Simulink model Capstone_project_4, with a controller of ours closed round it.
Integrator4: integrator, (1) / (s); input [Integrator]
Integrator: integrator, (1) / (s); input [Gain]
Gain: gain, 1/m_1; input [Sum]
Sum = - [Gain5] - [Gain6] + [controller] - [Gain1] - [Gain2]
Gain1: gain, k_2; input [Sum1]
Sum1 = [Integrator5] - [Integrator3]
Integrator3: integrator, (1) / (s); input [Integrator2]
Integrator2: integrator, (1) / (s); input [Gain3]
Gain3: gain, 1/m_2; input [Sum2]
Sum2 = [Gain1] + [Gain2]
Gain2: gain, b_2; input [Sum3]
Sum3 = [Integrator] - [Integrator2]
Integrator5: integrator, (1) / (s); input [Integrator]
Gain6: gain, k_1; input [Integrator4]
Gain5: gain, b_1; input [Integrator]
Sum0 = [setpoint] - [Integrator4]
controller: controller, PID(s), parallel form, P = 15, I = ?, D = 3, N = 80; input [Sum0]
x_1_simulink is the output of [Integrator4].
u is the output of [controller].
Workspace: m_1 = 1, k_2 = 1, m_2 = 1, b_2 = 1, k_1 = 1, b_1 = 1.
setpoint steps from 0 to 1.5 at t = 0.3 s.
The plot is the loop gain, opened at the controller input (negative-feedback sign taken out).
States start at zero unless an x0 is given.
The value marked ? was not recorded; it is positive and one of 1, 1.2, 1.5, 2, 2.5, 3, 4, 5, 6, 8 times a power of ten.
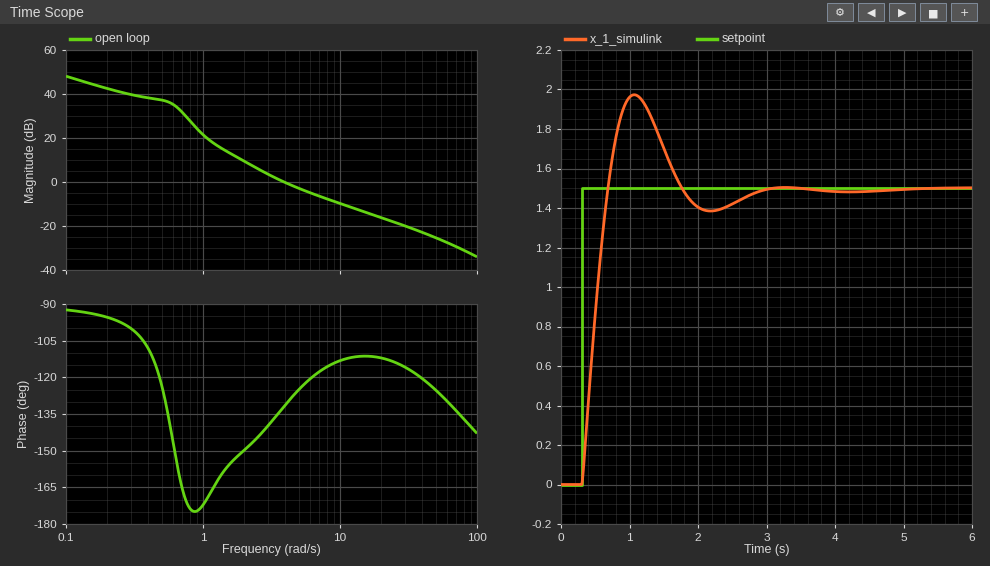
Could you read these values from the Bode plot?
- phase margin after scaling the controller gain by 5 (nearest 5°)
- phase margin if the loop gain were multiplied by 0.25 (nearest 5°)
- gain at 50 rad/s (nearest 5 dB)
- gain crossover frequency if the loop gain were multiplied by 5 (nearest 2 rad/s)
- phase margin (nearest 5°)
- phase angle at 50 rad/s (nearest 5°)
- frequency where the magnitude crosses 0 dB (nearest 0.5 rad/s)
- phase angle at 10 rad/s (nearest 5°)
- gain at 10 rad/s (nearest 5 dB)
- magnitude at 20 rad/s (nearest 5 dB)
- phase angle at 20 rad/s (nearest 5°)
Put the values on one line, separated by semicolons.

70°; 25°; -25 dB; 16 rad/s; 50°; -125°; 4.0 rad/s; -115°; -10 dB; -15 dB; -110°
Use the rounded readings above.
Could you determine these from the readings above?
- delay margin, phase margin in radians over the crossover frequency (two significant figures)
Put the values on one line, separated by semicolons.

0.22 s
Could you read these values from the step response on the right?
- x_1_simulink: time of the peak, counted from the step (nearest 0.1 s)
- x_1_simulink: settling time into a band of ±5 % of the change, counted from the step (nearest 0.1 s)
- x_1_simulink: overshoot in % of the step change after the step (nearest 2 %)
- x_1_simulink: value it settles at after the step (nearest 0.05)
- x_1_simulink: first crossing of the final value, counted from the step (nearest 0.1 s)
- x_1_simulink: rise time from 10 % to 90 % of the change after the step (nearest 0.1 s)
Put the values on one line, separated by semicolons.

0.8 s; 2.2 s; 32 %; 1.50; 0.4 s; 0.3 s
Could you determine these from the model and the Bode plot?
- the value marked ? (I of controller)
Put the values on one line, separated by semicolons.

25
